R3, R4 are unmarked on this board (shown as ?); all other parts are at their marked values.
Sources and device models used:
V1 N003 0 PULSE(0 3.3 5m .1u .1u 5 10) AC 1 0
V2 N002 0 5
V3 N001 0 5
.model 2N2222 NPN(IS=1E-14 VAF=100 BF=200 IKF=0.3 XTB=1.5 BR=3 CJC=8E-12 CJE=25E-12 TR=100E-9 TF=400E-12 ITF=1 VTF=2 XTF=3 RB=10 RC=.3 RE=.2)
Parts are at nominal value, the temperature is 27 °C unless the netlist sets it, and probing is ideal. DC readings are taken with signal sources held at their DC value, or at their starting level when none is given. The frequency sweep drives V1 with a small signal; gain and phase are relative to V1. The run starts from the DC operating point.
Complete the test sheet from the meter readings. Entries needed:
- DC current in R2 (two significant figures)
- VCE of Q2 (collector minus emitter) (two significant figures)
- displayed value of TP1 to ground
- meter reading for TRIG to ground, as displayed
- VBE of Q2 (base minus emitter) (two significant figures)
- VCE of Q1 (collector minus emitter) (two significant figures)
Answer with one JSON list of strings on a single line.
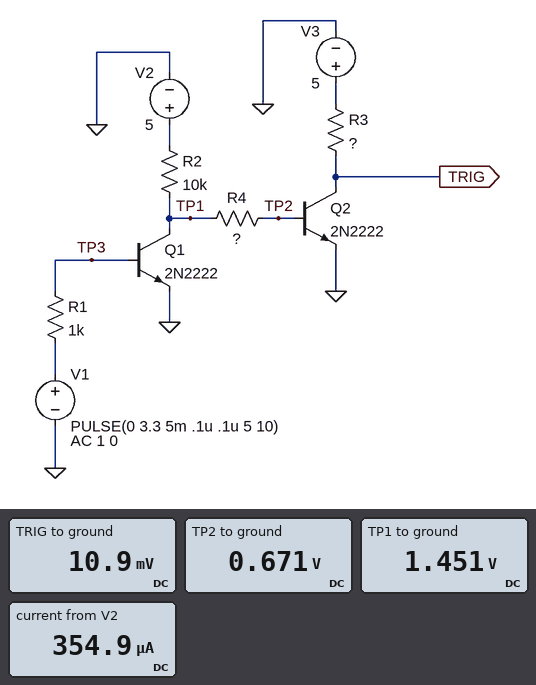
["350 µA", "11 mV", "1.451 V", "10.9 mV", "670 mV", "1.5 V"]
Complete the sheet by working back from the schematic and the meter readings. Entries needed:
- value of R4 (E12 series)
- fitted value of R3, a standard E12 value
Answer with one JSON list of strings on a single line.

["2.2 kΩ", "27 kΩ"]
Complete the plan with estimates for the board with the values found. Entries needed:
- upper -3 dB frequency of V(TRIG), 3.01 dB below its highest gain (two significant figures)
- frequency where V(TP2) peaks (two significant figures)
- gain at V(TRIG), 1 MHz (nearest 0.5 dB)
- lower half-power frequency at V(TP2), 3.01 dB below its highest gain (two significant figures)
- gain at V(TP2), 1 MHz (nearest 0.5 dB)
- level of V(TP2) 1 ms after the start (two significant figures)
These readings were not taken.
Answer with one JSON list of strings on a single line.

["28 MHz", "9.5 MHz", "-67.5 dB", "3.0 MHz", "-58.5 dB", "670 mV"]
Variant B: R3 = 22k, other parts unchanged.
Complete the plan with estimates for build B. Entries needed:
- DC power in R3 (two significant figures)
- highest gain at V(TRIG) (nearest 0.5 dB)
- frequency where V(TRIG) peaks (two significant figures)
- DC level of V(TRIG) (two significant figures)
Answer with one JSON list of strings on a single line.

["1.1 mW", "-55.0 dB", "9.9 MHz", "12 mV"]
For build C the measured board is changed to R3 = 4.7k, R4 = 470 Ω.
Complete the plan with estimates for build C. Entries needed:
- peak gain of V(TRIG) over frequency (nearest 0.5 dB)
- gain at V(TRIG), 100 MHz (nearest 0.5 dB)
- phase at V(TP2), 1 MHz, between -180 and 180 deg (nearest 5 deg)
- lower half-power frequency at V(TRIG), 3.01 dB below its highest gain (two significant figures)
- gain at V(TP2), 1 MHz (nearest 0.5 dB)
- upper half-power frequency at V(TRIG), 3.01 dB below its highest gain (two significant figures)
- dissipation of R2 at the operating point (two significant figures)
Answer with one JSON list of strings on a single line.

["-55.5 dB", "-60.5 dB", "55 deg", "4.0 MHz", "-59.5 dB", "71 MHz", "1.7 mW"]
